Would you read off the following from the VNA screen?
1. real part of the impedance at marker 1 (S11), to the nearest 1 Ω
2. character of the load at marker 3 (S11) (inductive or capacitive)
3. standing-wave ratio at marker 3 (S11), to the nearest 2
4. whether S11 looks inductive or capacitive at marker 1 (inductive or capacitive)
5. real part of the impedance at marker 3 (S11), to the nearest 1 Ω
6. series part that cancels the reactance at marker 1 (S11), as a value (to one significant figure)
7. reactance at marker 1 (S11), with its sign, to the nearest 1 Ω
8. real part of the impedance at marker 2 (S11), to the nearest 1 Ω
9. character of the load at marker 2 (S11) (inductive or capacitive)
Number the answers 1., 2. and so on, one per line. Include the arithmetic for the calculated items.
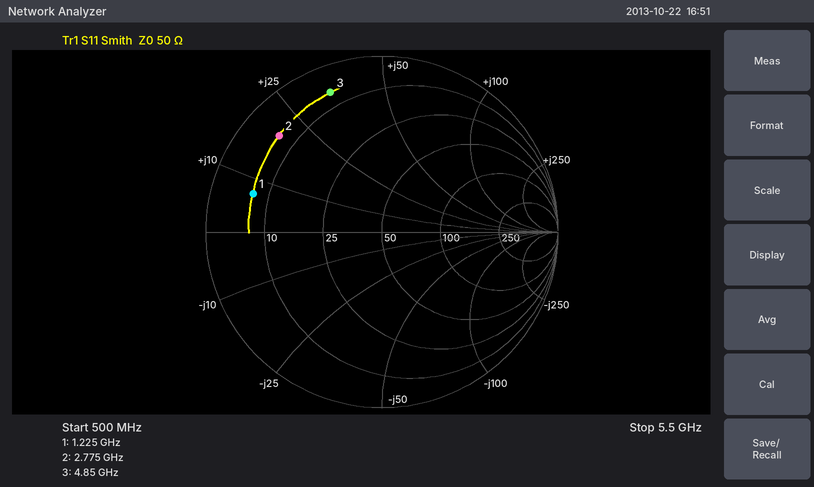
1. 7 Ω
2. inductive
3. 12
4. inductive
5. 6 Ω
6. C = 1/(2π × 1.225 GHz × 7 Ω) ≈ 18.6 pF, so 20 pF to one significant figure
7. +7 Ω
8. 6 Ω
9. inductive
